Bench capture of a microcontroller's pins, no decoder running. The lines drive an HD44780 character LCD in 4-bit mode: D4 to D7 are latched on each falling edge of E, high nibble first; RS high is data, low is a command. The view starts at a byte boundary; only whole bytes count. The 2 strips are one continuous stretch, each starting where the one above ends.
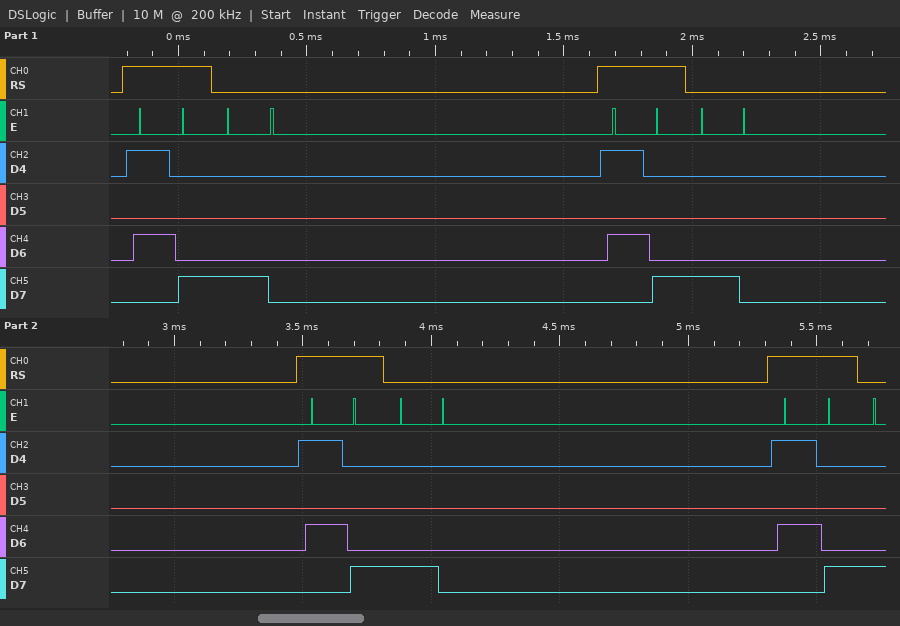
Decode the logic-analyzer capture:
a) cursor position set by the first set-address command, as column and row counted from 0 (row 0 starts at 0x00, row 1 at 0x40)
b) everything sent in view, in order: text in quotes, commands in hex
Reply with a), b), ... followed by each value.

a) column 0, row 0
b) "X" 0x80 "X" 0x80 "X" 0x80 "X"
